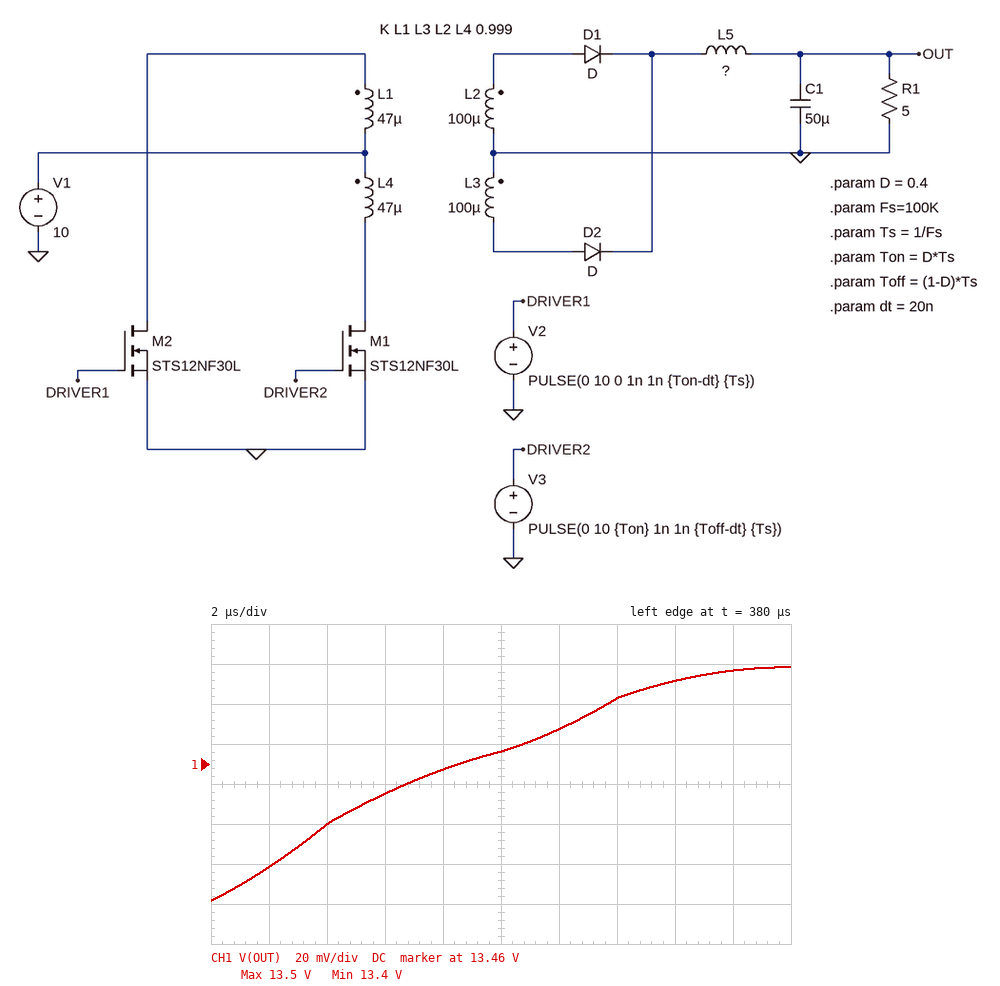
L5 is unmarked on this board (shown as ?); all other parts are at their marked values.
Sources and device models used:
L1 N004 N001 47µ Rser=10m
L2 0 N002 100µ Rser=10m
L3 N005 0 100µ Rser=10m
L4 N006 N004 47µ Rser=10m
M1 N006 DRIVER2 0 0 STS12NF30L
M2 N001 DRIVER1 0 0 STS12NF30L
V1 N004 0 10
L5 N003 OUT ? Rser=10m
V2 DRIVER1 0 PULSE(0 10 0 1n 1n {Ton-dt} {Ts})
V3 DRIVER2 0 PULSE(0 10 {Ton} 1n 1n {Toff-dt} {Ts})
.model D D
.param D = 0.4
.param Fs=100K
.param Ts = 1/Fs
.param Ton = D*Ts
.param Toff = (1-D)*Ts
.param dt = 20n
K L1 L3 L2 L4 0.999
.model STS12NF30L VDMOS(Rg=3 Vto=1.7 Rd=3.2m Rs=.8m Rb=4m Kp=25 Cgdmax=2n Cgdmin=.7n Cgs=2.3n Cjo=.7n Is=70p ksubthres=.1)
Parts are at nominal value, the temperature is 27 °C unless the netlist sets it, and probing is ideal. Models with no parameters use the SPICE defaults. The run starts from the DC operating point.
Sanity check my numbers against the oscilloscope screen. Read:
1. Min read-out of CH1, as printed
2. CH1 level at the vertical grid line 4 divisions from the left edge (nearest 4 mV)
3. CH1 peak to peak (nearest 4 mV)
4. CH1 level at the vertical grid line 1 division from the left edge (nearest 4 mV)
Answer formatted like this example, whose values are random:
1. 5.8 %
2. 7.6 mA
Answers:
1. 13.4 V
2. 13.456 V
3. 116 mV
4. 13.408 V
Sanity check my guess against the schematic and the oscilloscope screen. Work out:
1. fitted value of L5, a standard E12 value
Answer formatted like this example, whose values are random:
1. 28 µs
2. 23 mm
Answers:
1. 8.2 µH
